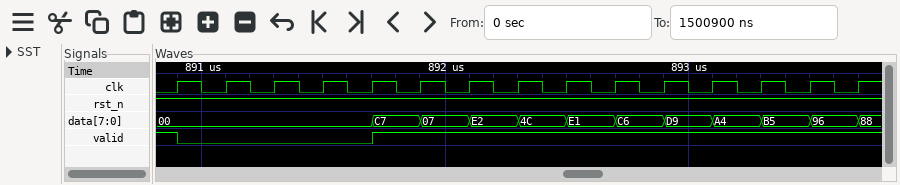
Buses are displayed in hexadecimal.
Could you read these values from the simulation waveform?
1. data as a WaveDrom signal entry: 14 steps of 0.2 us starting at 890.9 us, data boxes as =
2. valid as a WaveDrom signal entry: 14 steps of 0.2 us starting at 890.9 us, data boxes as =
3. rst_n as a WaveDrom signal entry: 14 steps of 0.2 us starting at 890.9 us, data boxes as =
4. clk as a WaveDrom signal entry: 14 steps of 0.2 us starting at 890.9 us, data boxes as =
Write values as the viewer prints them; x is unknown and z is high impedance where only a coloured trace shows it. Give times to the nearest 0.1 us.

{name: 'data', wave: '=...==========', data: '00 C7 07 E2 4C E1 C6 D9 A4 B5 96'}
{name: 'valid', wave: '0...1.........'}
{name: 'rst_n', wave: '1.............'}
{name: 'clk', wave: 'p.............'}
